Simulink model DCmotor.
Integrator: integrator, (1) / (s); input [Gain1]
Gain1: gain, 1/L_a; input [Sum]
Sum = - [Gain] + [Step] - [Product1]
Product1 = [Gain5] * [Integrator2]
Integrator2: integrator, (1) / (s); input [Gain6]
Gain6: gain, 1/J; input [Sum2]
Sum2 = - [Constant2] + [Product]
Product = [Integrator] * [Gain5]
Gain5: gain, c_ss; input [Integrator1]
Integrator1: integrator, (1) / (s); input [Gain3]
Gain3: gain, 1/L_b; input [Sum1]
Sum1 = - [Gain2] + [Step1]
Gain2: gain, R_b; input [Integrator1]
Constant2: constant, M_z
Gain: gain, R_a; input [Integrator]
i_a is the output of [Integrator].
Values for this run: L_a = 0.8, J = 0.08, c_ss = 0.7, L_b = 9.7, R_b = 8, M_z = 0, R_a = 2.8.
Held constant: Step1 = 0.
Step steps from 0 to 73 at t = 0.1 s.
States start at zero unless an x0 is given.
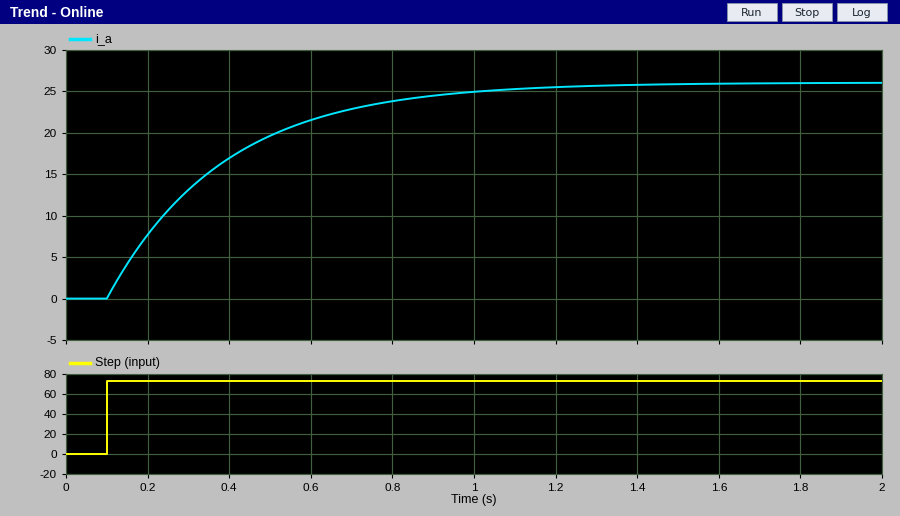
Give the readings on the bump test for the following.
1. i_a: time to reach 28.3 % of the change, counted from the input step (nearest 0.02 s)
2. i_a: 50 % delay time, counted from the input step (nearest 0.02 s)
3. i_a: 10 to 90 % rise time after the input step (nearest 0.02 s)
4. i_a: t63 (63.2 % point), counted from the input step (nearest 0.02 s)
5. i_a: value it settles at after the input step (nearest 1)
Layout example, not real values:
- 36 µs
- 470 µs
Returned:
- 0.10 s
- 0.20 s
- 0.62 s
- 0.28 s
- 26
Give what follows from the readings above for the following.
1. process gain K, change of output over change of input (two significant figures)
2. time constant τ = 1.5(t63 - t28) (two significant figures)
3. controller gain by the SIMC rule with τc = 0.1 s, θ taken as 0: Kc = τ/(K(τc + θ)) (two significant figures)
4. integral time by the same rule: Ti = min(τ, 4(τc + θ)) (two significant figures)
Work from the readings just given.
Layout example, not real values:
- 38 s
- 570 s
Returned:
- 0.36
- 0.27 s
- 7.5
- 0.27 s
